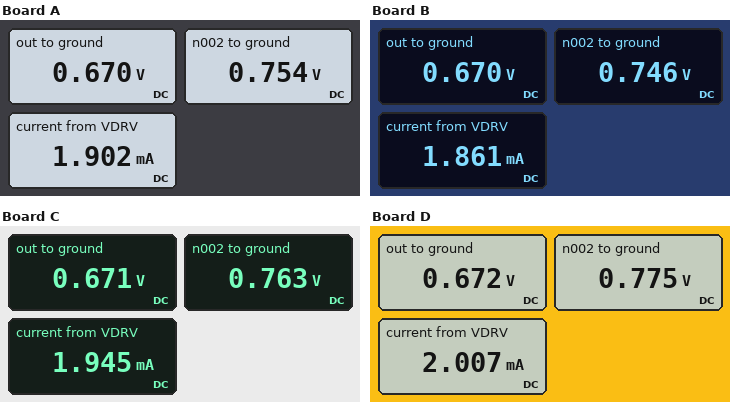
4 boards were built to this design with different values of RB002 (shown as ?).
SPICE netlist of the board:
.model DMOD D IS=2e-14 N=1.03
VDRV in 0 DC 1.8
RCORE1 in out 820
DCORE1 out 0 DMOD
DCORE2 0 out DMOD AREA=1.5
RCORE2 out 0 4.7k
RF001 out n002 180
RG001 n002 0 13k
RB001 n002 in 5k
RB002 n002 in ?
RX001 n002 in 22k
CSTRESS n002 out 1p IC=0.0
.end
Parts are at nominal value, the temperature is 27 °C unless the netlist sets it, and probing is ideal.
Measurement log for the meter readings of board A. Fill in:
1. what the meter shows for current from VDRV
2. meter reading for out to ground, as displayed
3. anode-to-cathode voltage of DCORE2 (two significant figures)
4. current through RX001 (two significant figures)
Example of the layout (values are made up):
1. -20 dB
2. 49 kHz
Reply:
1. 1.902 mA
2. 0.670 V
3. -670 mV
4. 48 µA
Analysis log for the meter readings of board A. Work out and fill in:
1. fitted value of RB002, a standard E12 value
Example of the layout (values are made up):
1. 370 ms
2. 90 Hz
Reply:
1. 3.9 kΩ
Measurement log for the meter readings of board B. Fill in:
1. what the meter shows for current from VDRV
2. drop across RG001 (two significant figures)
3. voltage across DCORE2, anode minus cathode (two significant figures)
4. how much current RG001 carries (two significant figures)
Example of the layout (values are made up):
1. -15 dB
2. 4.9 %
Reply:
1. 1.861 mA
2. 750 mV
3. -670 mV
4. 57 µA
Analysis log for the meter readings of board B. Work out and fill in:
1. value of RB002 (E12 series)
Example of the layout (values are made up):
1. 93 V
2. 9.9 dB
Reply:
1. 4.7 kΩ
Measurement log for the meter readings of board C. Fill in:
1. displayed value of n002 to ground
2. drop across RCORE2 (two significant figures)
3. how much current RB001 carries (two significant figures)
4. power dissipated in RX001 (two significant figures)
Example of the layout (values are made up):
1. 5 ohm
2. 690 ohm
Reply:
1. 0.763 V
2. 670 mV
3. 210 µA
4. 49 µW
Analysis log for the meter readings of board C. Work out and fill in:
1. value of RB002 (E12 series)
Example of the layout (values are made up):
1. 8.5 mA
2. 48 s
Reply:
1. 3.3 kΩ
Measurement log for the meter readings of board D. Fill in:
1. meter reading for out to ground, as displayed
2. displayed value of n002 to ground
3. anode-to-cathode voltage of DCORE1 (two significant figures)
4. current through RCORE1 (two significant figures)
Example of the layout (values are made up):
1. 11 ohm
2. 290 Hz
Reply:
1. 0.672 V
2. 0.775 V
3. 670 mV
4. 1.4 mA
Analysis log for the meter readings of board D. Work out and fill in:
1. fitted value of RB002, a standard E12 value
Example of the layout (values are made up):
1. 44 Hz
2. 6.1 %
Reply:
1. 2.7 kΩ
